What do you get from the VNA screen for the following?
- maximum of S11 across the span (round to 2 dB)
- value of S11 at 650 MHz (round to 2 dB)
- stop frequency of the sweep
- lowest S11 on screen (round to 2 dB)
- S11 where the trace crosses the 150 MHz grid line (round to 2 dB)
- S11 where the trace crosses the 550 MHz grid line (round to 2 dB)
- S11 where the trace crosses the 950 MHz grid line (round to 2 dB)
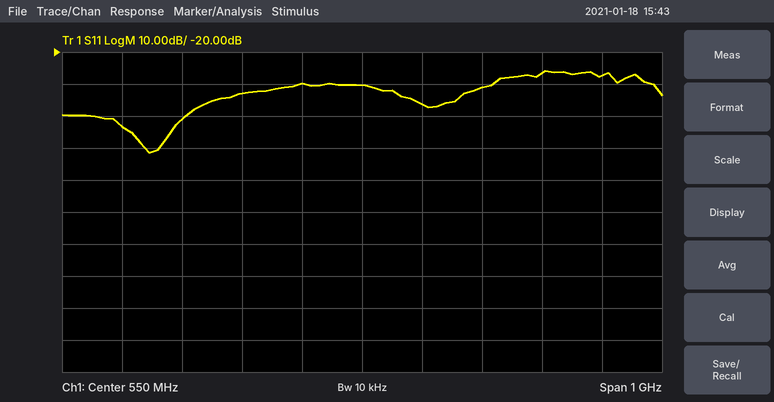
-26 dB
-36 dB
1.05 GHz
-52 dB
-44 dB
-30 dB
-28 dB
